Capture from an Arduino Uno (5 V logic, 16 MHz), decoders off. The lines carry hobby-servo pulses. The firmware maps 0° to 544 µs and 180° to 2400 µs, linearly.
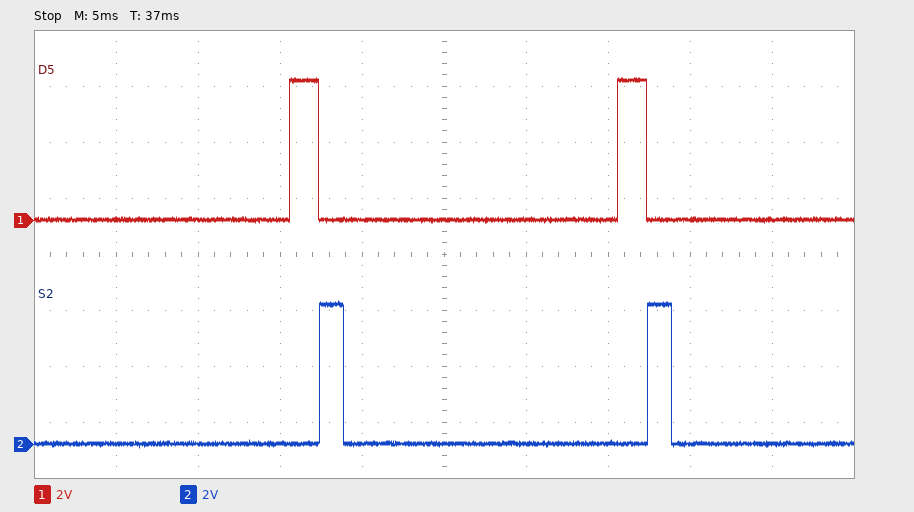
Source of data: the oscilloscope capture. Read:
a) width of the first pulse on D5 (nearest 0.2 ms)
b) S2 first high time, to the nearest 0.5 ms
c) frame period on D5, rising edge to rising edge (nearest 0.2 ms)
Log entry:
1.8 ms
1.5 ms
20.0 ms
